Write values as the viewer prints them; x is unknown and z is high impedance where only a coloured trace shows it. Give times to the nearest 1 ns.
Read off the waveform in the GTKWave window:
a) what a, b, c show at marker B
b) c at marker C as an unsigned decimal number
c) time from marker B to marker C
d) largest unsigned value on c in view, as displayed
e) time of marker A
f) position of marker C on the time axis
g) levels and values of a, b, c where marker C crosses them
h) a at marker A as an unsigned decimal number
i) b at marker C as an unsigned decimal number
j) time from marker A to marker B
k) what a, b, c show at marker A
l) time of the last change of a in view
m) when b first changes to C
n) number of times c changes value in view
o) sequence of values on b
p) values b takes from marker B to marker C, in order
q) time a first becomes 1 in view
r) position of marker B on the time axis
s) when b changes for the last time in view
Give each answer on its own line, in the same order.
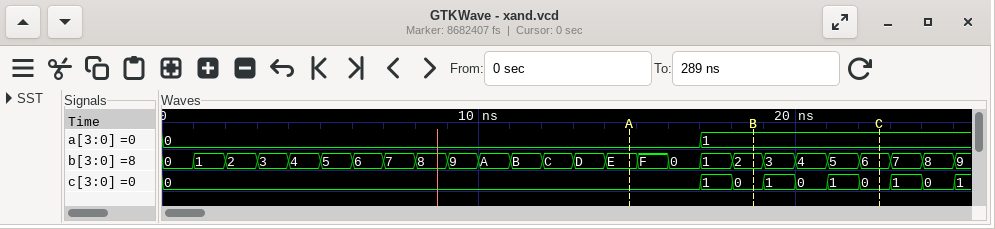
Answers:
a=1, b=2, c=0
0
4 ns
1
15 ns
23 ns
a=1, b=6, c=0
0
6
4 ns
a=0, b=E, c=0
17 ns
12 ns
9
0, 1, 2, 3, 4, 5, 6, 7, 8, 9, A, B, C, D, E, F, 0, 1, 2, 3, 4, 5, 6, 7, 8, 9
2, 3, 4, 5, 6
17 ns
19 ns
25 ns
